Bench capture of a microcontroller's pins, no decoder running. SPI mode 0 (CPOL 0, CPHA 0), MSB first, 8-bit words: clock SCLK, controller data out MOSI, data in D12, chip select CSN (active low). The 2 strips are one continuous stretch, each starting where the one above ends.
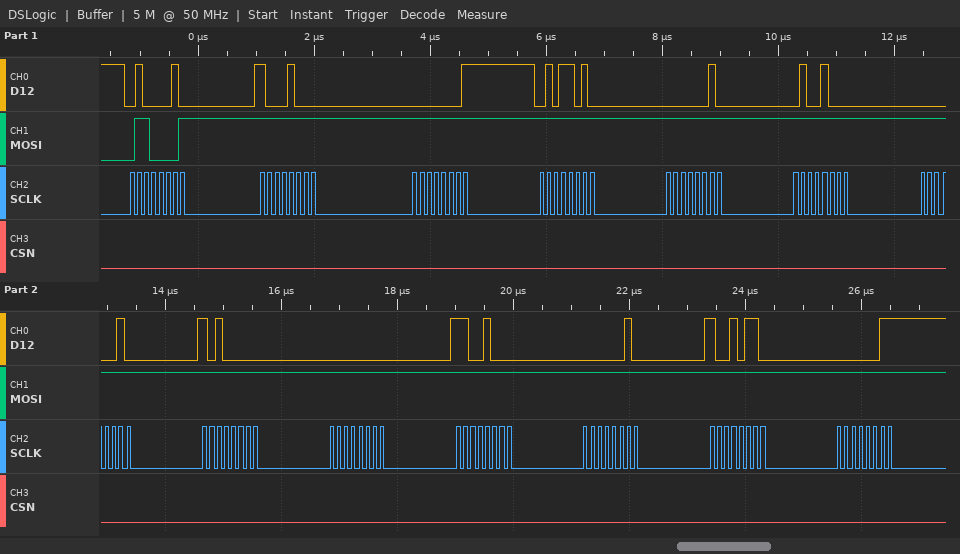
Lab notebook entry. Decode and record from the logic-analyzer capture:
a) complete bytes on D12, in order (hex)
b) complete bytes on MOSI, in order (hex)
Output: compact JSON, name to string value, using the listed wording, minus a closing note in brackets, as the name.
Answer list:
{"complete bytes on D12, in order": "42 88 01 5A 02 48 02 A0 00 C8 02 96 03", "complete bytes on MOSI, in order": "61 FF FF FF FF FF FF FF FF FF FF FF FF"}
